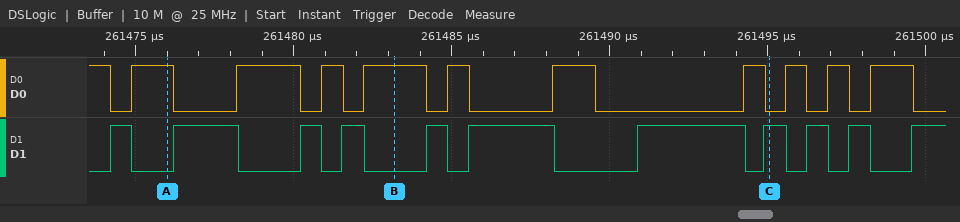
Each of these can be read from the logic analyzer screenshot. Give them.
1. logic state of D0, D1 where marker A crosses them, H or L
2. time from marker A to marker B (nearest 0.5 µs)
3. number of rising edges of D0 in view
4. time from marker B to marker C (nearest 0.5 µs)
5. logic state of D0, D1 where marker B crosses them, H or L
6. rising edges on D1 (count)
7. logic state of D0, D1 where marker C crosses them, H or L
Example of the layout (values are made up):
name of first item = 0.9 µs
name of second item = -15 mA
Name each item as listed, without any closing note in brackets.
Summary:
logic state of D0, D1 where marker A crosses them, H or L = D0=H, D1=L
time from marker A to marker B = 7 µs
number of rising edges of D0 in view = 10
time from marker B to marker C = 12 µs
logic state of D0, D1 where marker B crosses them, H or L = D0=H, D1=L
rising edges on D1 = 11
logic state of D0, D1 where marker C crosses them, H or L = D0=L, D1=H
